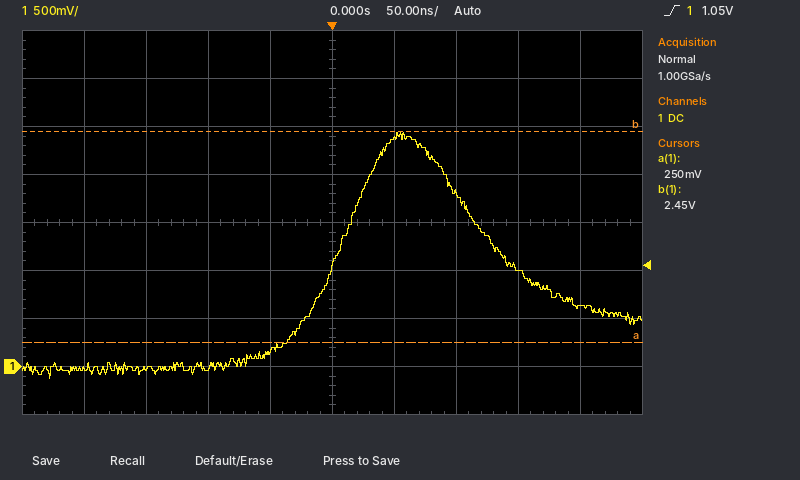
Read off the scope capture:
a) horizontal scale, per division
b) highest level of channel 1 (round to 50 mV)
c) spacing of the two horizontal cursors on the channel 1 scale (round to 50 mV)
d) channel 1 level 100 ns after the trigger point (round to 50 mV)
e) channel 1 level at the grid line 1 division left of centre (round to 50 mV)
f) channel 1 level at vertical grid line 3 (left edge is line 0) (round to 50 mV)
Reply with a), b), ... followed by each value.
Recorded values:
a) 50 ns
b) 2.45 V
c) 2.20 V
d) 1.80 V
e) 150 mV
f) 0 mV
